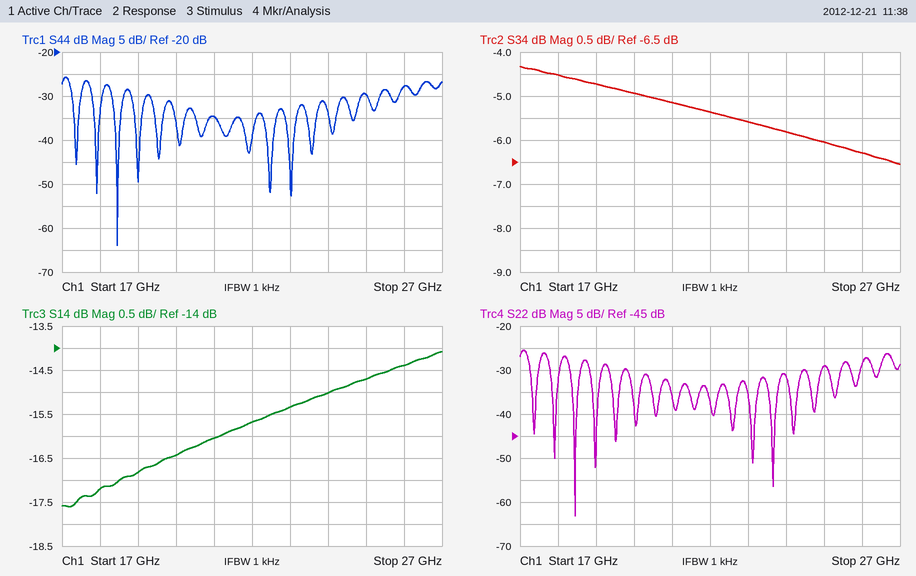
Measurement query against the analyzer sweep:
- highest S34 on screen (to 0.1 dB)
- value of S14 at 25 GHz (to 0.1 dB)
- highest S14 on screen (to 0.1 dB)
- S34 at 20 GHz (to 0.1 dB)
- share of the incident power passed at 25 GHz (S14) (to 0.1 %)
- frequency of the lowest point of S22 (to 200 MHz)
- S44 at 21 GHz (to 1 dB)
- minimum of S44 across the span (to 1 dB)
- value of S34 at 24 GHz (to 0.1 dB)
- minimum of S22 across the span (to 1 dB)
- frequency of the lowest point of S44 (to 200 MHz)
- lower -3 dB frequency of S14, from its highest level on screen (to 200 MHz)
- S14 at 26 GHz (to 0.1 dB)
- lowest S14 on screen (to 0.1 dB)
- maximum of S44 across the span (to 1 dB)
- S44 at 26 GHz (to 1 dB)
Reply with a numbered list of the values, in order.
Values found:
1. -4.3 dB
2. -14.7 dB
3. -14.1 dB
4. -4.9 dB
5. 3.4 %
6. 18.4 GHz
7. -35 dB
8. -64 dB
9. -5.8 dB
10. -63 dB
11. 18.4 GHz
12. 18.4 GHz
13. -14.4 dB
14. -17.6 dB
15. -26 dB
16. -28 dB
